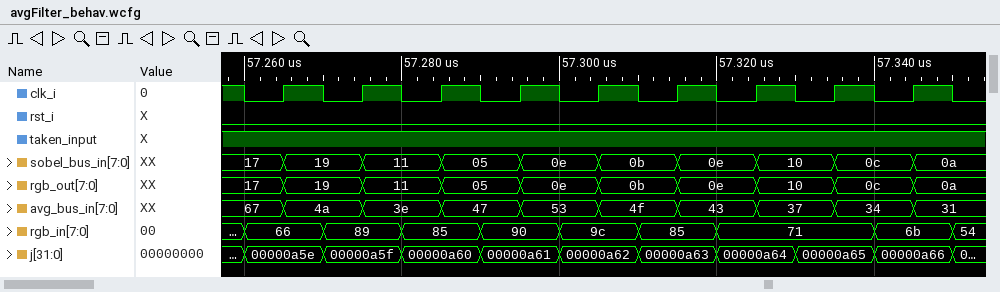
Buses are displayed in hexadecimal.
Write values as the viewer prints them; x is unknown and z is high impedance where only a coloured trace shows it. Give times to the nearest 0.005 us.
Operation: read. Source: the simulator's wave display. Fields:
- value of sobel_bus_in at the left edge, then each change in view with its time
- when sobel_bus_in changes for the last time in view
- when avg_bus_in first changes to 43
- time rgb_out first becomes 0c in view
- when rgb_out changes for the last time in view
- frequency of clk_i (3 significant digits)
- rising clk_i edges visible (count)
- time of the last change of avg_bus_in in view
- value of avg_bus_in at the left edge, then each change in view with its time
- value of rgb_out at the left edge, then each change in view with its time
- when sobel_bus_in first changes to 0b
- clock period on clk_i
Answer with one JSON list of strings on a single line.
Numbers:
["17, 19 at 57.265 us, 11 at 57.275 us, 05 at 57.285 us, 0e at 57.295 us, 0b at 57.305 us, 0e at 57.315 us, 10 at 57.325 us, 0c at 57.335 us, 0a at 57.345 us", "57.345 us", "57.315 us", "57.335 us", "57.345 us", "100 MHz", "9", "57.345 us", "67, 4a at 57.265 us, 3e at 57.275 us, 47 at 57.285 us, 53 at 57.295 us, 4f at 57.305 us, 43 at 57.315 us, 37 at 57.325 us, 34 at 57.335 us, 31 at 57.345 us", "17, 19 at 57.265 us, 11 at 57.275 us, 05 at 57.285 us, 0e at 57.295 us, 0b at 57.305 us, 0e at 57.315 us, 10 at 57.325 us, 0c at 57.335 us, 0a at 57.345 us", "57.305 us", "0.01 us"]
